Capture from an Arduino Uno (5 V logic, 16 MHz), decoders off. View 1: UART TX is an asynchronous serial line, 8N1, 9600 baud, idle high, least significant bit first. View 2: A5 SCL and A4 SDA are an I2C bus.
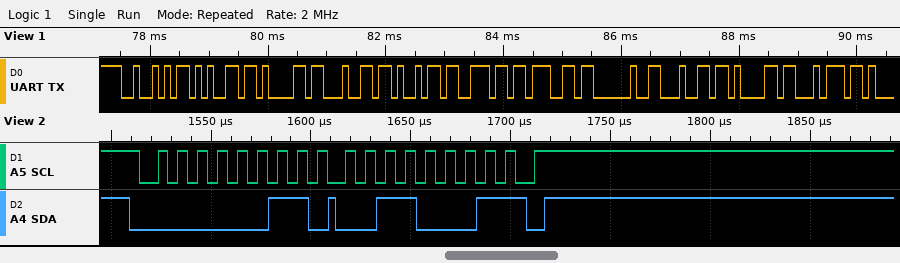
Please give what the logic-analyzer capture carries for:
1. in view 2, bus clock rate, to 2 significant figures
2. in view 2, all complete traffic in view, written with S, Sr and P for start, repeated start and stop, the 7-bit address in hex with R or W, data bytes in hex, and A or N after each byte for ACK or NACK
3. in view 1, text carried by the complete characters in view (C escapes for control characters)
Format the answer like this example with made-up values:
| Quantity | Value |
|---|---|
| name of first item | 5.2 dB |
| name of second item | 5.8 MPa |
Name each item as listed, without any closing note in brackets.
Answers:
| Quantity | Value |
|---|---|
| in view 2, bus clock rate, to 2 significant figures | 100 kHz |
| in view 2, all complete traffic in view, written with S, Sr and P for start, repeated start and stop, the 7-bit address in hex with R or W, data bytes in hex, and A or N after each byte for ACK or NACK | S 01R A 31 N P |
| in view 1, text carried by the complete characters in view | "Reading dat" |
